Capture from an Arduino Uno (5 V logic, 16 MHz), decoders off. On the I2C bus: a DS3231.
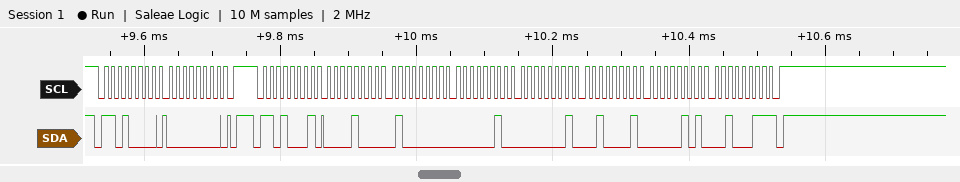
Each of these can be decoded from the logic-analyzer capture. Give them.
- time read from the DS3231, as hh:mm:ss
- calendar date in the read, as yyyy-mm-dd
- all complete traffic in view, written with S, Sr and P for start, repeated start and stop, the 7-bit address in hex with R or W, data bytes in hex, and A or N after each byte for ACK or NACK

02:40:08
2023-05-21
S 68W A 00 A P S 68R A 08 A 40 A 02 A 01 A 21 A 05 A 23 N P
